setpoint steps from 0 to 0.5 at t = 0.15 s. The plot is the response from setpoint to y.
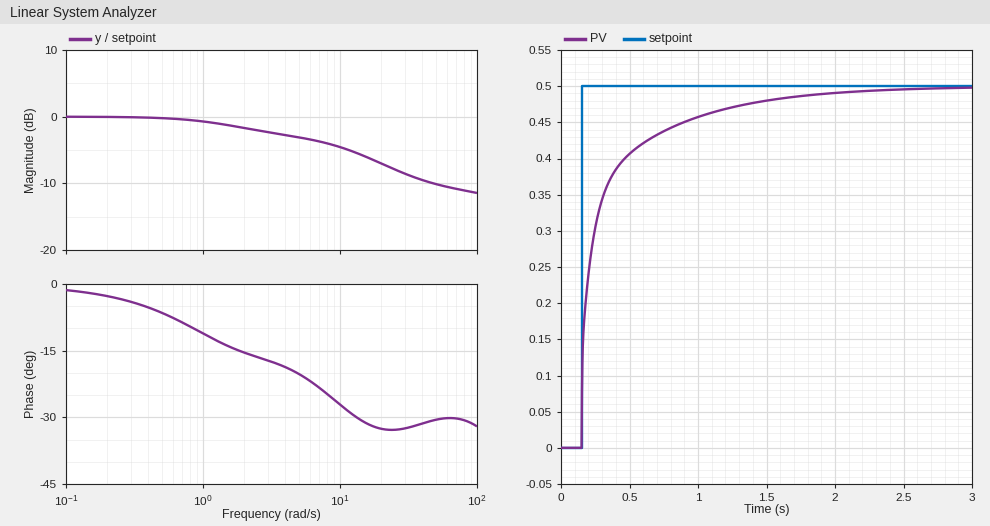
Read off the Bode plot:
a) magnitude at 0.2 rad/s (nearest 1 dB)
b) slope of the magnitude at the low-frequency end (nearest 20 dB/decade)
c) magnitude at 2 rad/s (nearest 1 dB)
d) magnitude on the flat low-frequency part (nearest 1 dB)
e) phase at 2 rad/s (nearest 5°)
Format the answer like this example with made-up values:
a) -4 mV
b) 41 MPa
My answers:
a) 0 dB
b) 0 dB/decade
c) -2 dB
d) 0 dB
e) -15°
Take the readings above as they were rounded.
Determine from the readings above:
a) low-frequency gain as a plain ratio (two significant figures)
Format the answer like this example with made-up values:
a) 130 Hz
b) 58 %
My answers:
a) 1.0
